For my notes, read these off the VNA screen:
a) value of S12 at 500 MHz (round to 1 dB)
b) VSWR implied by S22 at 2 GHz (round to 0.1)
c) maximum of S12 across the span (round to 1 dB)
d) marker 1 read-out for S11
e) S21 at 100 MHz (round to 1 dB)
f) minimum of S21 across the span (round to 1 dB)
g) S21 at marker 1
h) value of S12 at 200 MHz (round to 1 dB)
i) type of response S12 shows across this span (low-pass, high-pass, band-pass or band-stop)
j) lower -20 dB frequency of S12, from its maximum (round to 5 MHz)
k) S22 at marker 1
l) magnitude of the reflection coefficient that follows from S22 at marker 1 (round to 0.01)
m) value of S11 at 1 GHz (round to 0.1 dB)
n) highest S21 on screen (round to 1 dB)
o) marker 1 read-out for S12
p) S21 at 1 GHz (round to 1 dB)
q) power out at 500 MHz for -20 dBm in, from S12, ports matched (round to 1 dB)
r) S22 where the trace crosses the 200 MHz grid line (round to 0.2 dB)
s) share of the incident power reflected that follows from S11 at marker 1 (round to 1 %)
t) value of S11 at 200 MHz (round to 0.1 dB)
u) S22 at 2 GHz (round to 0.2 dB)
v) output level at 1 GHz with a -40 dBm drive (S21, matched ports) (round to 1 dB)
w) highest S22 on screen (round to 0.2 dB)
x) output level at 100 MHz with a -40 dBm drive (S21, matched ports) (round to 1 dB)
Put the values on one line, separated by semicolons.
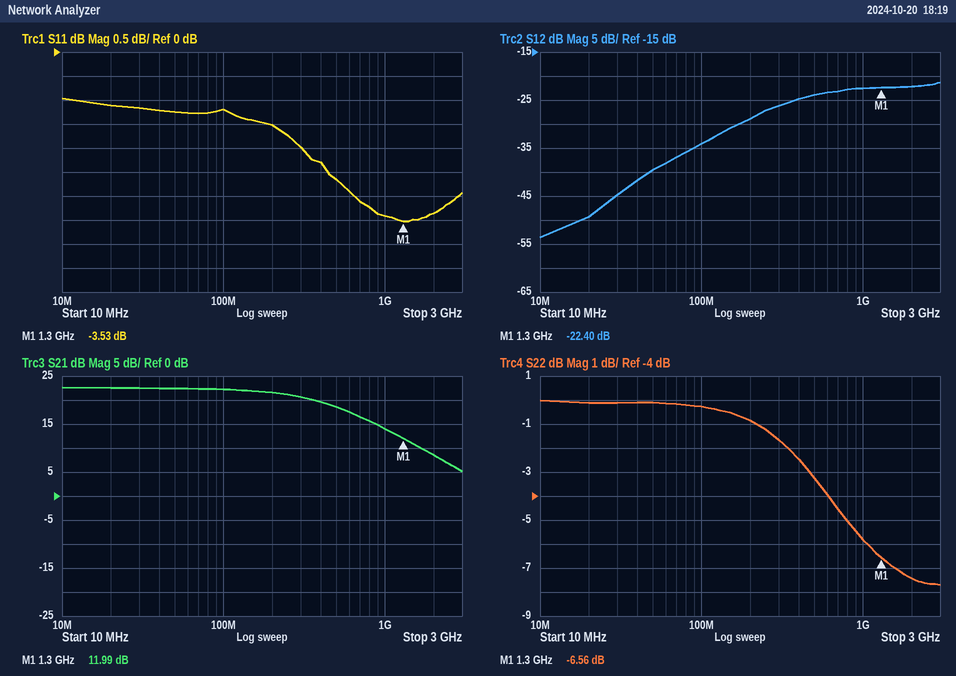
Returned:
-24 dB; 2.5; -21 dB; -3.53 dB; 22 dB; 5 dB; 11.99 dB; -29 dB; high-pass; 40 MHz; -6.56 dB; 0.47; -3.4 dB; 23 dB; -22.40 dB; 14 dB; -44 dBm; -0.8 dB; 44 %; -1.5 dB; -7.4 dB; -26 dBm; 0.0 dB; -18 dBm
